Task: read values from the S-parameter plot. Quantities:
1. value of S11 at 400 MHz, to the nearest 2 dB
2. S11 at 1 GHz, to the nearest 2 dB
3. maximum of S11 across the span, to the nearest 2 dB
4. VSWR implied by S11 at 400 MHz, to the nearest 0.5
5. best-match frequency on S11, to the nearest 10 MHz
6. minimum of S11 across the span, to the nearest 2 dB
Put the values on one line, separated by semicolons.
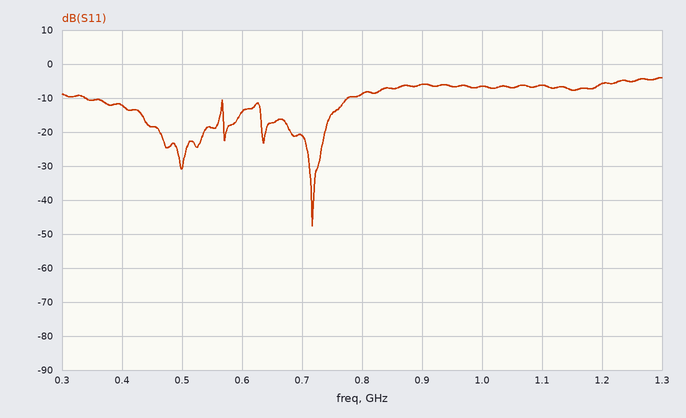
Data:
-12 dB; -6 dB; -4 dB; 1.5; 720 MHz; -48 dB
